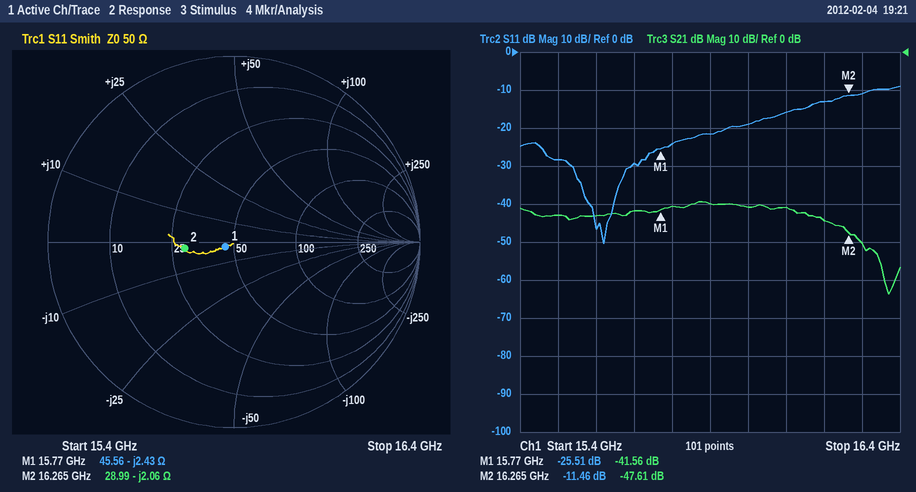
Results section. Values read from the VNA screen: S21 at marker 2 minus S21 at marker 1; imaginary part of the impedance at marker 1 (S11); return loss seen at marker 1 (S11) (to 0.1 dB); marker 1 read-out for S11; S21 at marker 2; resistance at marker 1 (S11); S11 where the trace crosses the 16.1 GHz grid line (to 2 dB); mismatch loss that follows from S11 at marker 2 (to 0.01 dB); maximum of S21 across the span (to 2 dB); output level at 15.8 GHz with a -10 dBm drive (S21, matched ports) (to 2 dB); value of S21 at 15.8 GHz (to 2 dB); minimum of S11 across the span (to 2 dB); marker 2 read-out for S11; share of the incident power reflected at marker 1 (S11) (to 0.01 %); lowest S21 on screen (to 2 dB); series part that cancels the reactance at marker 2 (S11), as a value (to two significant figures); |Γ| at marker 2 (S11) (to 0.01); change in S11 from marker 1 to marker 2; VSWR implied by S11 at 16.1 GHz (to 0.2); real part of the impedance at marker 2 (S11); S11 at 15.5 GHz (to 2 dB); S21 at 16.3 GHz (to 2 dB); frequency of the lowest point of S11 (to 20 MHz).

-6.05 dB
-2.43 Ω
25.5 dB
-25.51 dB
-47.61 dB
45.56 Ω
-16 dB
0.32 dB
-40 dB
-50 dBm
-40 dB
-50 dB
-11.46 dB
0.28 %
-64 dB
20 pH
0.27
14.05 dB
1.4
28.99 Ω
-28 dB
-50 dB
15.62 GHz
